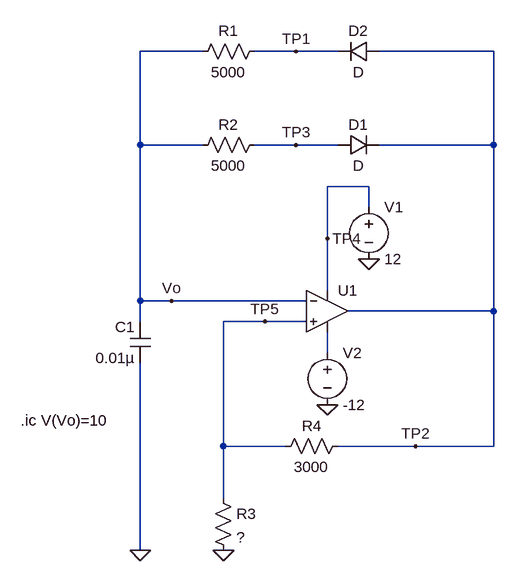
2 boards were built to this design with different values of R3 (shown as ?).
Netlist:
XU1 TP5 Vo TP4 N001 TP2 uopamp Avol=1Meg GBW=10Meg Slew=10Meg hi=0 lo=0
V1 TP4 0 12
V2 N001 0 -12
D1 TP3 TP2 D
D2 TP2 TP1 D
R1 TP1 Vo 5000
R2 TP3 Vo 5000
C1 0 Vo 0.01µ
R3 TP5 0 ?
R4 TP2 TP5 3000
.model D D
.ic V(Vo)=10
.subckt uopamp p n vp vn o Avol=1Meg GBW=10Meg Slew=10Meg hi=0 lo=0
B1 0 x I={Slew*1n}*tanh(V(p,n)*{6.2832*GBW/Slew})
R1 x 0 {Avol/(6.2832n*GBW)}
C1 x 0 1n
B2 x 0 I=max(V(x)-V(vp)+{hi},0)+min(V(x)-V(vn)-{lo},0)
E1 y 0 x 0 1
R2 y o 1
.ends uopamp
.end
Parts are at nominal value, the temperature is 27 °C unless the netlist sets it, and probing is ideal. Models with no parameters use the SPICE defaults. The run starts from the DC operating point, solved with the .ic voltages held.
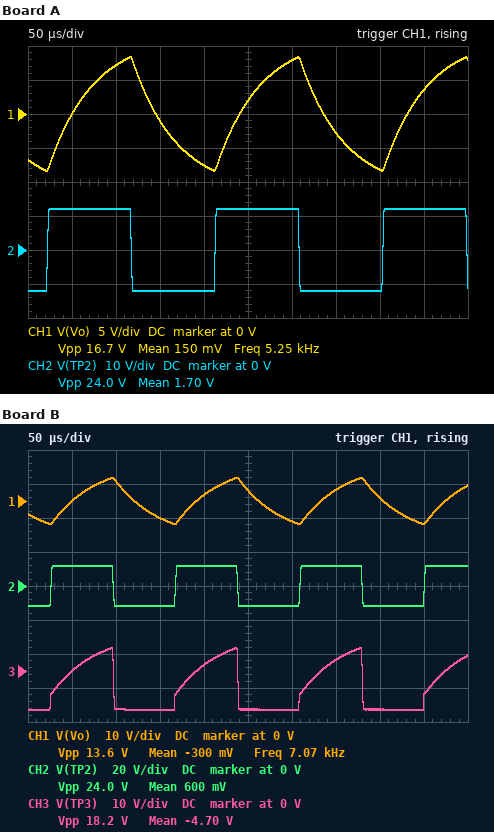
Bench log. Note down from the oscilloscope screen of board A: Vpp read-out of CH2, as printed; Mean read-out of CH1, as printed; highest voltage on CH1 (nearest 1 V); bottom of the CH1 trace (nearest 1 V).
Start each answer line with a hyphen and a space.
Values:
- 24.0 V
- 150 mV
- 8 V
- -8 V
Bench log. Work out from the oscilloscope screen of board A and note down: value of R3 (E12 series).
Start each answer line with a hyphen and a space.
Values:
- 6.8 kΩ
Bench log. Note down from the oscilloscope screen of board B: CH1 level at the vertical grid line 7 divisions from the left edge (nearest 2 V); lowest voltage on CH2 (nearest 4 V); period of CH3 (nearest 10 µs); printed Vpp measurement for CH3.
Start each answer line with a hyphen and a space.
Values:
- 4 V
- -12 V
- 140 µs
- 18.2 V
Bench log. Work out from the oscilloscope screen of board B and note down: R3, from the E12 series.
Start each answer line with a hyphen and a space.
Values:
- 3.9 kΩ
